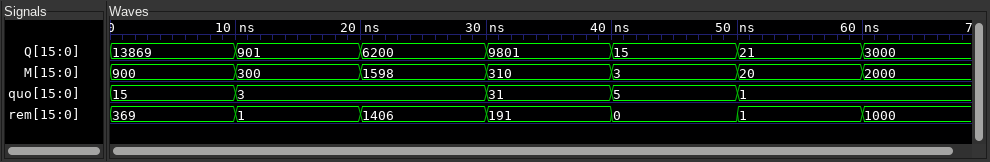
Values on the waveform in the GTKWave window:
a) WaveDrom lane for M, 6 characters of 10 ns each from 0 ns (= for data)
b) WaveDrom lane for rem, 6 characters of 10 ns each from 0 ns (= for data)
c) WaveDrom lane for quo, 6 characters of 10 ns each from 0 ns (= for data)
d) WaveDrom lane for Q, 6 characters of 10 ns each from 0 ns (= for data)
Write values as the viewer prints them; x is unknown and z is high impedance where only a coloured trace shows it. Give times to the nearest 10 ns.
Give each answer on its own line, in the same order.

{name: 'M', wave: '======', data: '900 300 1598 310 3 20'}
{name: 'rem', wave: '======', data: '369 1 1406 191 0 1'}
{name: 'quo', wave: '==.===', data: '15 3 31 5 1'}
{name: 'Q', wave: '======', data: '13869 901 6200 9801 15 21'}
